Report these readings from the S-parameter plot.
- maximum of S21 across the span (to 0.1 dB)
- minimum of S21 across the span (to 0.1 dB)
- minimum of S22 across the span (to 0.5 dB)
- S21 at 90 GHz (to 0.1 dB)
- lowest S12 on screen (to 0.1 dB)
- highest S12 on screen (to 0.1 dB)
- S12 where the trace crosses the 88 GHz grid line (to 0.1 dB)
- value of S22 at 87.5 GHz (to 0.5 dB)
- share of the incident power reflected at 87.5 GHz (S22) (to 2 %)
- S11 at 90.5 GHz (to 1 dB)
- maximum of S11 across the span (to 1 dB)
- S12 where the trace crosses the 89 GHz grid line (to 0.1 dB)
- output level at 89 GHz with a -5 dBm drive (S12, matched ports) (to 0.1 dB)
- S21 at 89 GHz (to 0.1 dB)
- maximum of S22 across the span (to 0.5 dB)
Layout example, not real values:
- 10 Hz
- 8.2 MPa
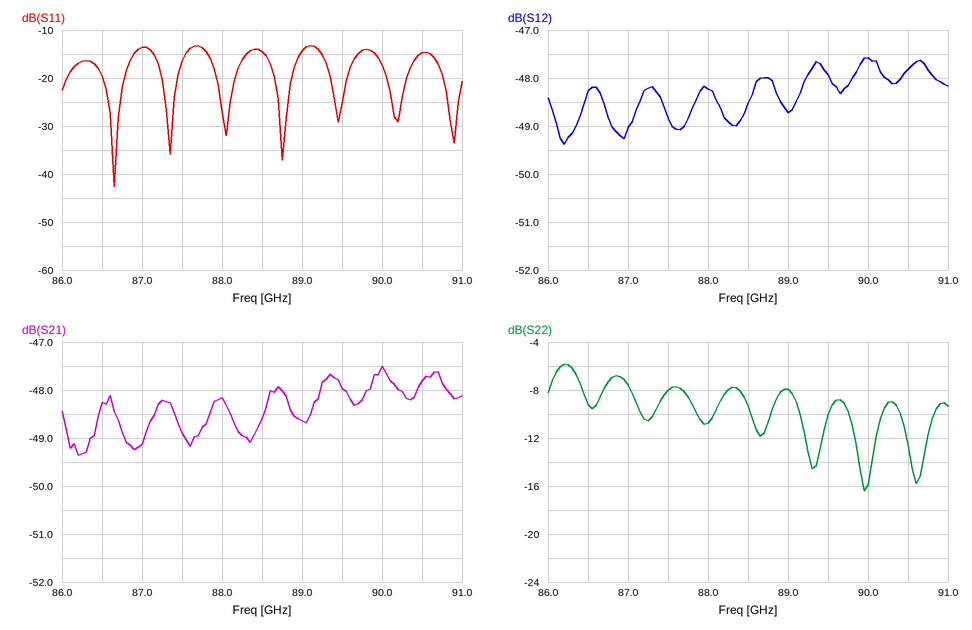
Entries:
- -47.5 dB
- -49.4 dB
- -16.5 dB
- -47.5 dB
- -49.4 dB
- -47.6 dB
- -48.2 dB
- -8.0 dB
- 16 %
- -15 dB
- -13 dB
- -48.7 dB
- -53.7 dBm
- -48.6 dB
- -6.0 dB
